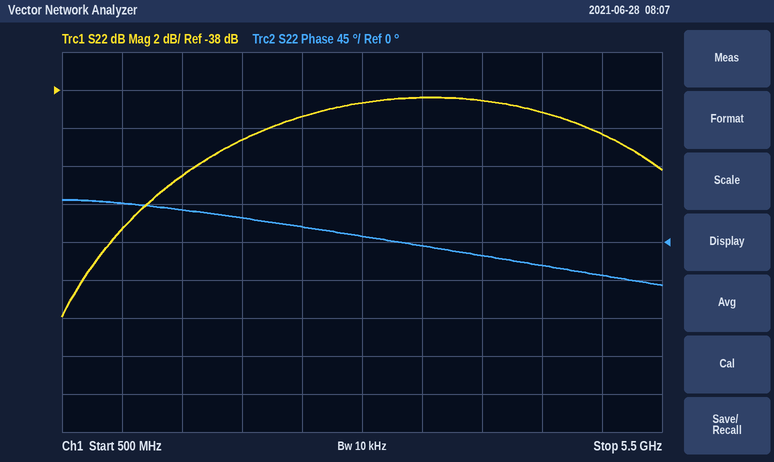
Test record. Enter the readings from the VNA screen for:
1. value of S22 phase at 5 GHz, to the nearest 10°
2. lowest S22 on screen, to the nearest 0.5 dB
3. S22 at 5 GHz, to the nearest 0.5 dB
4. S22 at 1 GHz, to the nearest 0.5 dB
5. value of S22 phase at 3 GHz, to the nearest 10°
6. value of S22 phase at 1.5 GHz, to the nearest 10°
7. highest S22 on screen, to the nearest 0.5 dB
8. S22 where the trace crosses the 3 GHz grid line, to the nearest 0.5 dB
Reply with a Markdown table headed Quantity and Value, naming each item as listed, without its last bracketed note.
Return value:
| Quantity | Value |
|---|---|
| value of S22 phase at 5 GHz, to the nearest 10° | -40° |
| lowest S22 on screen, to the nearest 0.5 dB | -50.0 dB |
| S22 at 5 GHz, to the nearest 0.5 dB | -40.5 dB |
| S22 at 1 GHz, to the nearest 0.5 dB | -45.5 dB |
| value of S22 phase at 3 GHz, to the nearest 10° | 10° |
| value of S22 phase at 1.5 GHz, to the nearest 10° | 40° |
| highest S22 on screen, to the nearest 0.5 dB | -38.5 dB |
| S22 where the trace crosses the 3 GHz grid line, to the nearest 0.5 dB | -38.5 dB |
